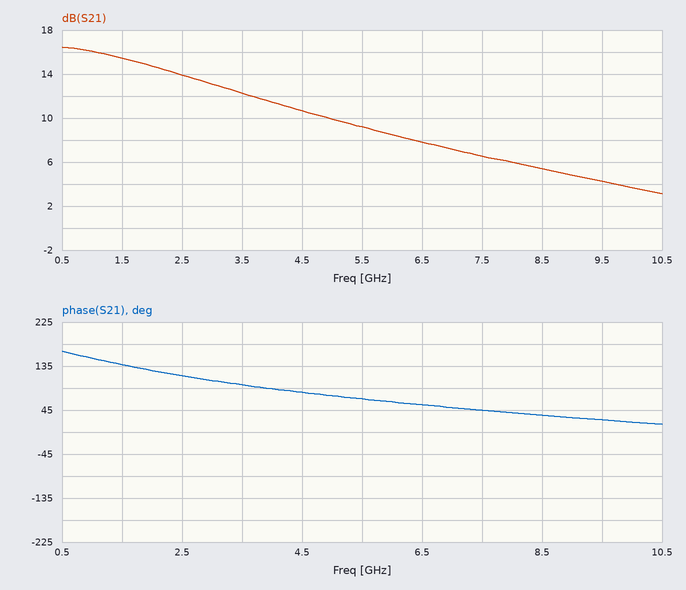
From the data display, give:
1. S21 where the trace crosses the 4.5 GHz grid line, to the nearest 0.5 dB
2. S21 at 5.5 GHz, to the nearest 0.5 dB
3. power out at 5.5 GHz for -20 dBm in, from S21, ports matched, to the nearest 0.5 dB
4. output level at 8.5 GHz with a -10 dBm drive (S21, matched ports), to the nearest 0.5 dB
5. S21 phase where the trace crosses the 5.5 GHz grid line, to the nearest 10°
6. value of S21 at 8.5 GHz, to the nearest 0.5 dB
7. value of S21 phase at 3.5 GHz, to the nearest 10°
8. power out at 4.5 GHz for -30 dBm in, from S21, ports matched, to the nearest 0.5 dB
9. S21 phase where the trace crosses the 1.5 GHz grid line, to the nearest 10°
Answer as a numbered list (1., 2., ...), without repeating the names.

1. 10.5 dB
2. 9.0 dB
3. -11.0 dBm
4. -4.5 dBm
5. 70°
6. 5.5 dB
7. 100°
8. -19.5 dBm
9. 140°
